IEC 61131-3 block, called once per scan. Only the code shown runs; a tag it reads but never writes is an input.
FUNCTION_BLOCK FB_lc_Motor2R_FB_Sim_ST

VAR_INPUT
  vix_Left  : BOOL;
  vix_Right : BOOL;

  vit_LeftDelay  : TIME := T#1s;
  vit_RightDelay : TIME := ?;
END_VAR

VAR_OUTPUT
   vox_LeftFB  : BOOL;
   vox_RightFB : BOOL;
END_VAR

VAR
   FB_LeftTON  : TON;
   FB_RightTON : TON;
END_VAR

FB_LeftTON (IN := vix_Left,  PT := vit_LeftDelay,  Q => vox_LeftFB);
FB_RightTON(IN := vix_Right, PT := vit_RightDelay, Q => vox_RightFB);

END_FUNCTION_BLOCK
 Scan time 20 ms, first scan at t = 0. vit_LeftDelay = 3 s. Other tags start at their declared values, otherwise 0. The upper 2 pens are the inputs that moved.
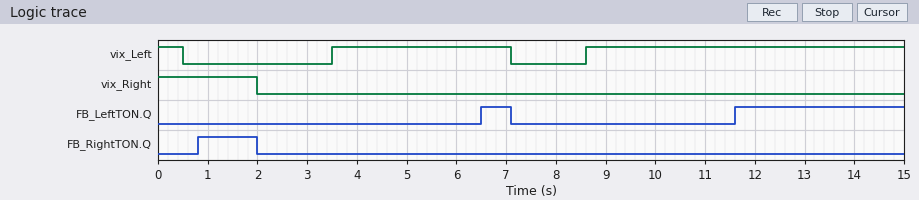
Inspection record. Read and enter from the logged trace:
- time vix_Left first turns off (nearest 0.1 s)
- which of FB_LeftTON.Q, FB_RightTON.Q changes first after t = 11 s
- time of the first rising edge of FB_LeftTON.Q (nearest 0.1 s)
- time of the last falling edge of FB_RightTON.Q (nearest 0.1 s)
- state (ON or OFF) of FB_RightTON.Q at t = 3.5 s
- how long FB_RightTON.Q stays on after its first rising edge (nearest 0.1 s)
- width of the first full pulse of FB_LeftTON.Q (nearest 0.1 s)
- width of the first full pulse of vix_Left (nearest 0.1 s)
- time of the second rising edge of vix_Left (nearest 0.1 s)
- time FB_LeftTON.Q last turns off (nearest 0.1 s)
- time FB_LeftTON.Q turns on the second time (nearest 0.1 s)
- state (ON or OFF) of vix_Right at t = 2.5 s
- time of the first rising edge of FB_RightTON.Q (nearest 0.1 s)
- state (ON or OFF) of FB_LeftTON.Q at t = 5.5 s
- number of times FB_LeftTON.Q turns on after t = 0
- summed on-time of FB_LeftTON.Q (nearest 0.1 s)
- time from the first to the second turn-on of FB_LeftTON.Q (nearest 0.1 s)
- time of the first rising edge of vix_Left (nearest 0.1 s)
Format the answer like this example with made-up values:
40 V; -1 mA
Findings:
0.5 s; FB_LeftTON.Q; 6.5 s; 2.0 s; OFF; 1.2 s; 0.6 s; 3.6 s; 8.6 s; 7.1 s; 11.6 s; OFF; 0.8 s; OFF; 2; 4.0 s; 5.1 s; 3.5 s
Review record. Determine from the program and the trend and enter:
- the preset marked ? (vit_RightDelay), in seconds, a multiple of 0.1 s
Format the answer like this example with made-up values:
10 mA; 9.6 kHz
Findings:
0.8 s
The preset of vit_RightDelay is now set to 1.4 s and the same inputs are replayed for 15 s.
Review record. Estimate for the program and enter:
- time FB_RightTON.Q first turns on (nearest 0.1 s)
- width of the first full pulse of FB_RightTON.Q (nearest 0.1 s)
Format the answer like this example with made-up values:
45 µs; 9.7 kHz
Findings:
1.4 s; 0.6 s
